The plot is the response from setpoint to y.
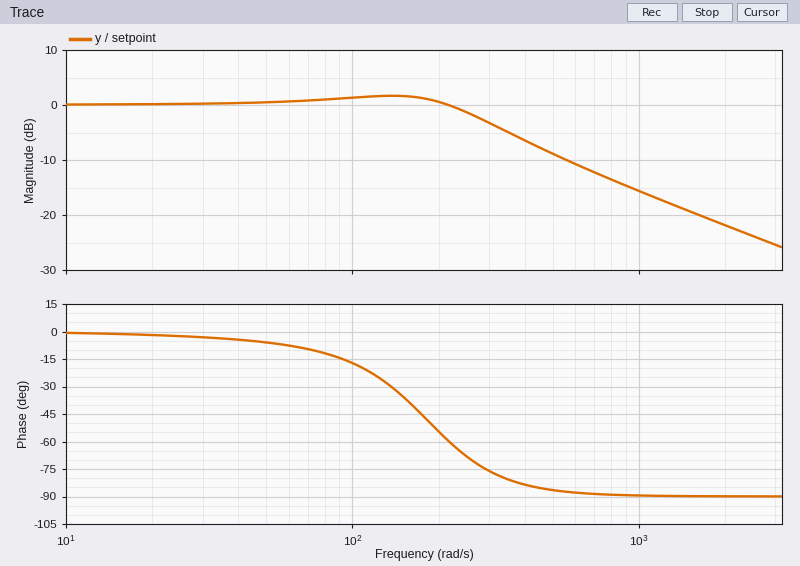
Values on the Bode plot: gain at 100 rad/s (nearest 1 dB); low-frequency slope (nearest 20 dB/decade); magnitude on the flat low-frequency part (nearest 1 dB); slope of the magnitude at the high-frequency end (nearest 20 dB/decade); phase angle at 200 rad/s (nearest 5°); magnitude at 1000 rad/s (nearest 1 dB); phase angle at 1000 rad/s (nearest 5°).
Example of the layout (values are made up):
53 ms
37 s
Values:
1 dB
0 dB/decade
0 dB
-20 dB/decade
-55°
-16 dB
-90°
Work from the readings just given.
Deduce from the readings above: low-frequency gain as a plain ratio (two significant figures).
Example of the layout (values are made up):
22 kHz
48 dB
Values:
1.0
